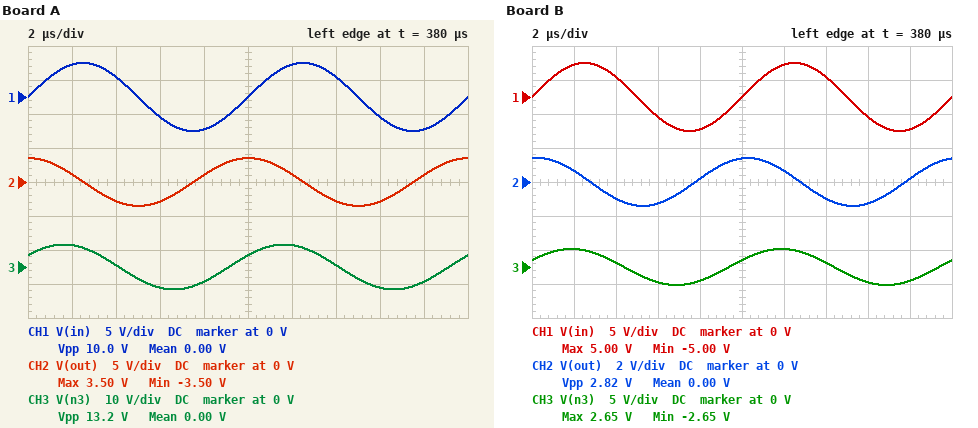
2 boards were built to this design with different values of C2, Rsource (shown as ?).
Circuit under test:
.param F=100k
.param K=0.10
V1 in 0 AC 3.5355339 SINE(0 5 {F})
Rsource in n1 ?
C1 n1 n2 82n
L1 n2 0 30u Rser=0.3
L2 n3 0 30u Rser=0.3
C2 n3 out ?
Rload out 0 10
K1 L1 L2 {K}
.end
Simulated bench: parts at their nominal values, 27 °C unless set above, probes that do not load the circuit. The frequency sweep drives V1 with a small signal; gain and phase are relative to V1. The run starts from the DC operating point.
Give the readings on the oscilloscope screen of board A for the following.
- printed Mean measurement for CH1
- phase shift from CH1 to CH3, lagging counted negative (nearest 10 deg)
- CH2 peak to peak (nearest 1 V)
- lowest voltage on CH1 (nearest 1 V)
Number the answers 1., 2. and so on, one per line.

1. 0.00 V
2. 30 deg
3. 7 V
4. -5 V
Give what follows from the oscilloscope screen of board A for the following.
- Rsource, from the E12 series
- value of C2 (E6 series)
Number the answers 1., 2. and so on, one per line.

1. 1.8 Ω
2. 100 nF
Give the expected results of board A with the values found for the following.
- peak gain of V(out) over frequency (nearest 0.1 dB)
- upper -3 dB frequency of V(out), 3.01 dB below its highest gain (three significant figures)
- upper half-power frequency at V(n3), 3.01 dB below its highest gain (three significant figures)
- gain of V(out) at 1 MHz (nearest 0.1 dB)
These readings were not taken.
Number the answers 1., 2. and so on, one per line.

1. -2.8 dB
2. 108 kHz
3. 108 kHz
4. -45.3 dB
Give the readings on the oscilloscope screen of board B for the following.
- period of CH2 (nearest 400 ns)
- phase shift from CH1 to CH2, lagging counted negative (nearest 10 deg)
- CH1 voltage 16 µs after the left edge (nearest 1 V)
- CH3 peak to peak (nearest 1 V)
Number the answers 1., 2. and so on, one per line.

1. 10.0 µs
2. 80 deg
3. -3 V
4. 5 V
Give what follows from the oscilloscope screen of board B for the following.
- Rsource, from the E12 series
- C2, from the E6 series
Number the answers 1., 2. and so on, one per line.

1. 5.6 Ω
2. 100 nF
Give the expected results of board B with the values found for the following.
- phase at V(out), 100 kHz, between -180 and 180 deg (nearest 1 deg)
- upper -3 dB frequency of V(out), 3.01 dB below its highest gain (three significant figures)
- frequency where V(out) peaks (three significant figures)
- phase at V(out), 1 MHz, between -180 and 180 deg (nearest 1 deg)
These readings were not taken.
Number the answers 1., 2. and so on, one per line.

1. 80 deg
2. 118 kHz
3. 102 kHz
4. -85 deg
